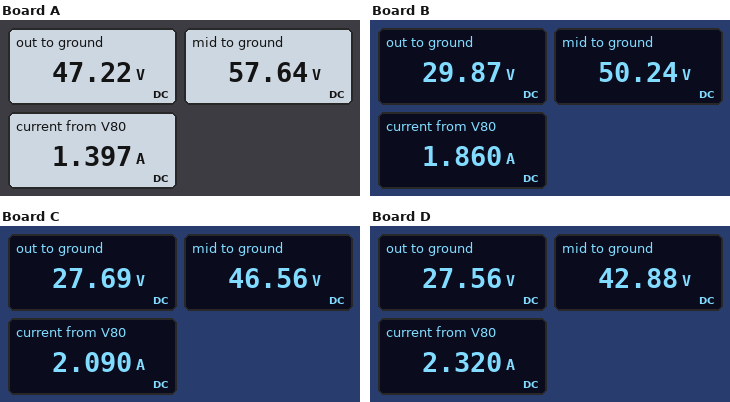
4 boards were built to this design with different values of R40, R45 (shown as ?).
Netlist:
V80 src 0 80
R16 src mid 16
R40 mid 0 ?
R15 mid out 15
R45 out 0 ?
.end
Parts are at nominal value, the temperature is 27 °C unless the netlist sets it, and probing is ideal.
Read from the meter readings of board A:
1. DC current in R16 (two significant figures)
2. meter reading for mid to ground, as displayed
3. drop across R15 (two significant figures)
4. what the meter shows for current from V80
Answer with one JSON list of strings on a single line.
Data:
["1.4 A", "57.64 V", "10 V", "1.397 A"]
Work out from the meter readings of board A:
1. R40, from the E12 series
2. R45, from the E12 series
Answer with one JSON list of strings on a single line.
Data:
["82 Ω", "68 Ω"]
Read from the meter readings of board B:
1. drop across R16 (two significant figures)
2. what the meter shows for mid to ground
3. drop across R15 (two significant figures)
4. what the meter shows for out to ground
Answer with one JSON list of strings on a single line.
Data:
["30 V", "50.24 V", "20 V", "29.87 V"]
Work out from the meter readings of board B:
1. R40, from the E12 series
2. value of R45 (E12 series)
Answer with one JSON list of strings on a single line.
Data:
["100 Ω", "22 Ω"]
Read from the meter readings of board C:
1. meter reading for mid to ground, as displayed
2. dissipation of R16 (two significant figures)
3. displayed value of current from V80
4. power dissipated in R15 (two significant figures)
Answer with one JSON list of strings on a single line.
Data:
["46.56 V", "70 W", "2.090 A", "24 W"]
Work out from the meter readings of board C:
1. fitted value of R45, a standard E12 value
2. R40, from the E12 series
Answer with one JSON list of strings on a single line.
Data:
["22 Ω", "56 Ω"]
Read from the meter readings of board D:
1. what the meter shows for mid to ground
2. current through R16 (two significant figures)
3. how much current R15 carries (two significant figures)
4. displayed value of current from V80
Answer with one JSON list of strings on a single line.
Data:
["42.88 V", "2.3 A", "1.0 A", "2.320 A"]
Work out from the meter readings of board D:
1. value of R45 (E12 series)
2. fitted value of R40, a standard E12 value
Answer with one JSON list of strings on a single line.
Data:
["27 Ω", "33 Ω"]
